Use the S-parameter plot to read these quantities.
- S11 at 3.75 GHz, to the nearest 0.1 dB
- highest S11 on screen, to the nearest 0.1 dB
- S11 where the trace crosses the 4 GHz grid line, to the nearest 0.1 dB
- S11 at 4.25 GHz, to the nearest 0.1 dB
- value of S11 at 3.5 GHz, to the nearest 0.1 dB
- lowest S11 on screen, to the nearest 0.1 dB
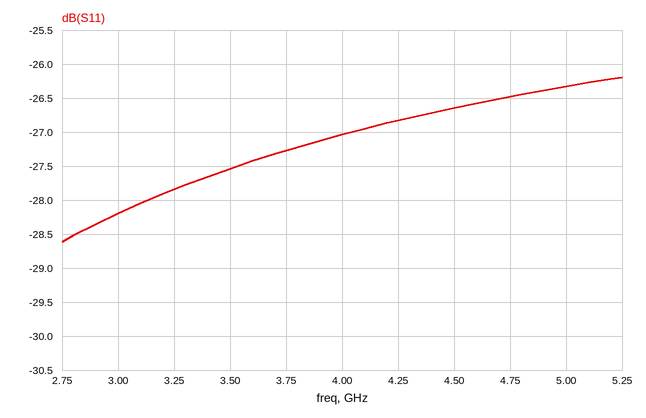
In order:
-27.3 dB
-26.2 dB
-27.0 dB
-26.8 dB
-27.5 dB
-28.6 dB
